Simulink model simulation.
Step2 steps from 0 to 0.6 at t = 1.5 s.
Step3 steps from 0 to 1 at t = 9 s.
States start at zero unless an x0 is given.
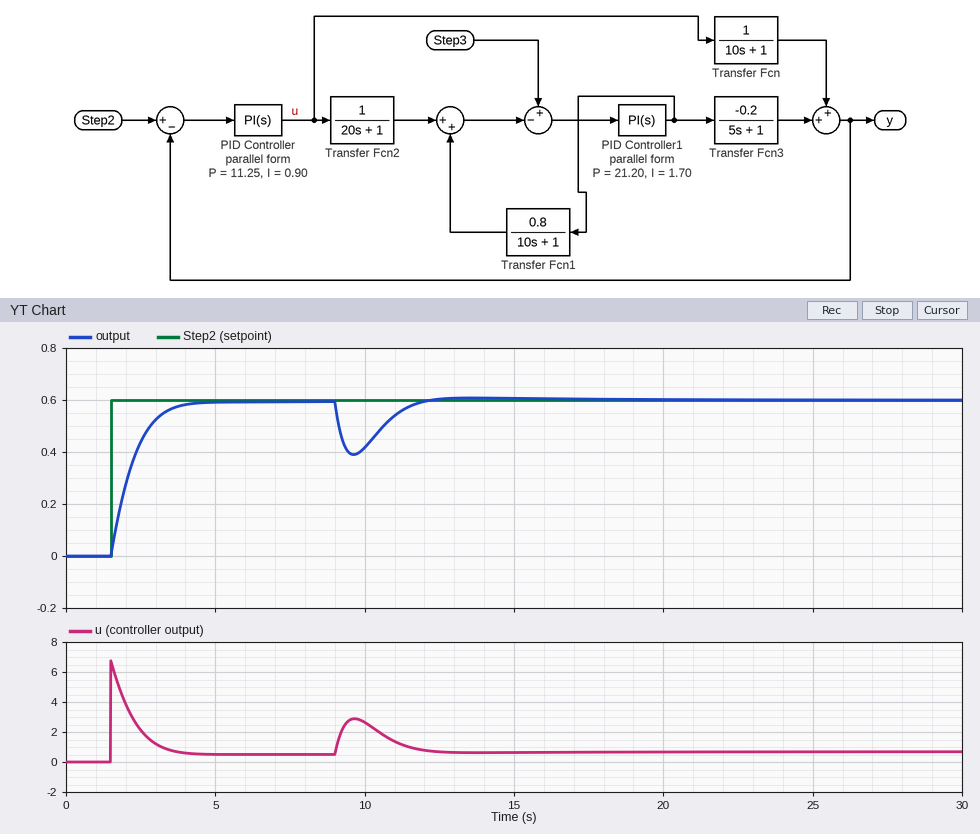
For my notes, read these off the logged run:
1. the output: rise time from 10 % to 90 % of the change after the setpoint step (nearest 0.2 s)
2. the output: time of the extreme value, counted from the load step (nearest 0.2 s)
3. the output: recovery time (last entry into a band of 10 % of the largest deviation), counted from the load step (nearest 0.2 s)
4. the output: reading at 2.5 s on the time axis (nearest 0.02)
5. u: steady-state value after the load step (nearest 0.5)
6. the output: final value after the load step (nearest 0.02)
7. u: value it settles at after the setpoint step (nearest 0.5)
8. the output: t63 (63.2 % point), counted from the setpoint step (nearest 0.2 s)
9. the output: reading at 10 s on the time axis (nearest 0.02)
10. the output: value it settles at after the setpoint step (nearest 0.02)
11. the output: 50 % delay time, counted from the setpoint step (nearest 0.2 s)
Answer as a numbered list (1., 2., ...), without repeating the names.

1. 1.6 s
2. 0.6 s
3. 2.6 s
4. 0.44
5. 0.5
6. 0.60
7. 0.5
8. 0.8 s
9. 0.42
10. 0.60
11. 0.6 s
